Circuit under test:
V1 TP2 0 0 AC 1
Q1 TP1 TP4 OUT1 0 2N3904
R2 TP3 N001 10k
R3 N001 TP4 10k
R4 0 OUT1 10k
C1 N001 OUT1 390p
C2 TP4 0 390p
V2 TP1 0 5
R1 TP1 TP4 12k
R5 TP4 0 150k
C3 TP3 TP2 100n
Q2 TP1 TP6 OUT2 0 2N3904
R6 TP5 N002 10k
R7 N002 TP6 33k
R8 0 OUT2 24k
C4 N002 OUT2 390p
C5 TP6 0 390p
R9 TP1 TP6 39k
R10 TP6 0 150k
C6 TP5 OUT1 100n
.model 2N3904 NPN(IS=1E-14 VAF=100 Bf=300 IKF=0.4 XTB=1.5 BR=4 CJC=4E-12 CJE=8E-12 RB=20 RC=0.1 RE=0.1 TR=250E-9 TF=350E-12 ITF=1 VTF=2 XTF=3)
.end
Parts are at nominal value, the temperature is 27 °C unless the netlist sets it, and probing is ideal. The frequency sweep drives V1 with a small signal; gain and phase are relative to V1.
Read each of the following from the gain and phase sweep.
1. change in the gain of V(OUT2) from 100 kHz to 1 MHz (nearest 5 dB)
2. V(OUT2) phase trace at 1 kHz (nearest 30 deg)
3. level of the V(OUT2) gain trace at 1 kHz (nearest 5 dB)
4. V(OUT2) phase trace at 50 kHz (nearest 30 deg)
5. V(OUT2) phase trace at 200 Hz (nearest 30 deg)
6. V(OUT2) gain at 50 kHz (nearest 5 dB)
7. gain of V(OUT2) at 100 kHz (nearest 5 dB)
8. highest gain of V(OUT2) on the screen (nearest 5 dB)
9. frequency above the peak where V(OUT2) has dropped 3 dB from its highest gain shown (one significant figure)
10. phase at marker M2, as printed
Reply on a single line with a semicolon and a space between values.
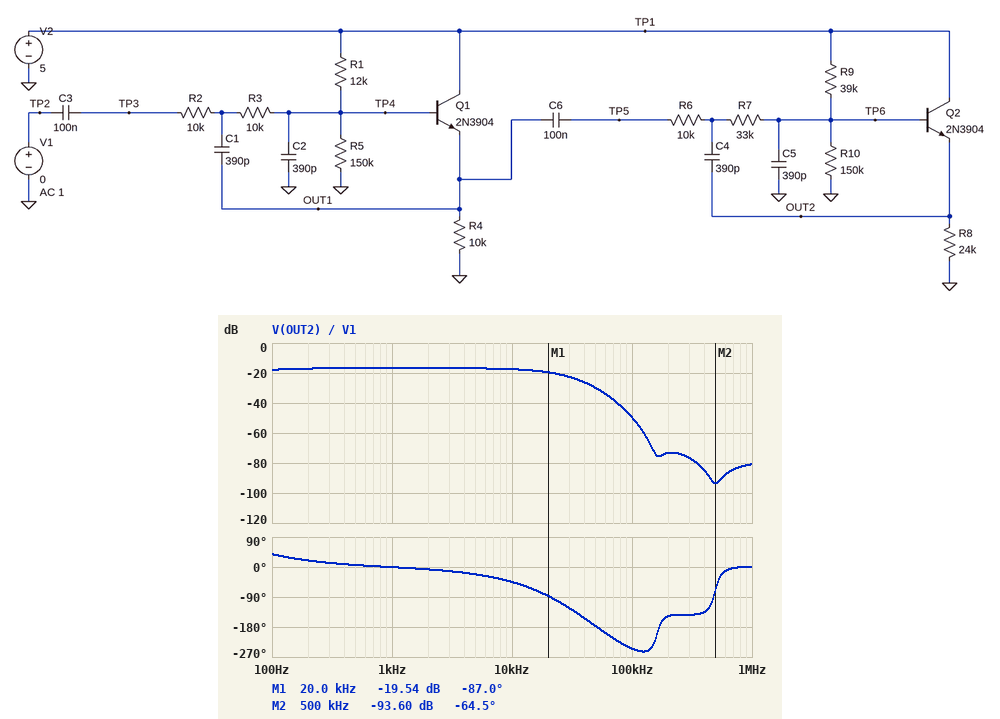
-30 dB; 0 deg; -15 dB; -180 deg; 30 deg; -30 dB; -50 dB; -15 dB; 20 kHz; -64.5 deg
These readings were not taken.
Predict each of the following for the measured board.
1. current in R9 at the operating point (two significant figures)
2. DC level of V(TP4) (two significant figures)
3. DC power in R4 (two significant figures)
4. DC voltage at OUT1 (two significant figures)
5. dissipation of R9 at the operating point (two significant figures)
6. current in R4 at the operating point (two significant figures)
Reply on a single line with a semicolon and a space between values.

27 µA; 4.6 V; 1.6 mW; 4.0 V; 28 µW; 400 µA
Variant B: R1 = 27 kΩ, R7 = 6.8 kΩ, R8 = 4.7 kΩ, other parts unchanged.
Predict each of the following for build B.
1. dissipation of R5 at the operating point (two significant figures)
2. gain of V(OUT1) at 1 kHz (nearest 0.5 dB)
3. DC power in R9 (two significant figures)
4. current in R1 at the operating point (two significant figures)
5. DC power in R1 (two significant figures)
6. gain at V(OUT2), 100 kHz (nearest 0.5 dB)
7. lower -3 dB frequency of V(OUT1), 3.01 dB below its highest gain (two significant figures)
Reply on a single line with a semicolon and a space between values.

120 µW; -5.5 dB; 31 µW; 29 µA; 23 µW; -33.0 dB; 37 Hz
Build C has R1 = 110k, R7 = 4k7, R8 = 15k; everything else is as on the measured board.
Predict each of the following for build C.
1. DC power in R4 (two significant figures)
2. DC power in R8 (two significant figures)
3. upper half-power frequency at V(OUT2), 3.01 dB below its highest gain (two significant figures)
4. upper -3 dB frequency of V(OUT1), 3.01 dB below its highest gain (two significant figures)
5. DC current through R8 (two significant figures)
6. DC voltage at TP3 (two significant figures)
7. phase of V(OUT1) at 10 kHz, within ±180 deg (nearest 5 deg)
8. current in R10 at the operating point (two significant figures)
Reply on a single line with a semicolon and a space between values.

490 µW; 740 µW; 26 kHz; 32 kHz; 220 µA; 2.8 V; -25 deg; 26 µA
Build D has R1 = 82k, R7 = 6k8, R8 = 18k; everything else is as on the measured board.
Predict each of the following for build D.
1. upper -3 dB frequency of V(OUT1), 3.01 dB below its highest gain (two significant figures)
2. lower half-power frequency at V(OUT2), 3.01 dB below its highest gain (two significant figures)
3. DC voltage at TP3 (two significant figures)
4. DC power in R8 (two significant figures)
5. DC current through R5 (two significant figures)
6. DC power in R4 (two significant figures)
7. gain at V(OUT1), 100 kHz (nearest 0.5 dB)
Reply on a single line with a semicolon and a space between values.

33 kHz; 43 Hz; 3.2 V; 620 µW; 21 µA; 660 µW; -18.0 dB
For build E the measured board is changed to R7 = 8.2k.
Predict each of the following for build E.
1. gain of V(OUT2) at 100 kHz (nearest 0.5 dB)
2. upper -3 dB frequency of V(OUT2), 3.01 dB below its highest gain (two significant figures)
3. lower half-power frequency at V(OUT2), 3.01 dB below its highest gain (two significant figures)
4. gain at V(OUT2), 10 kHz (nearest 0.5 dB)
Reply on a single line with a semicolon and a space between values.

-35.5 dB; 31 kHz; 65 Hz; -13.5 dB
